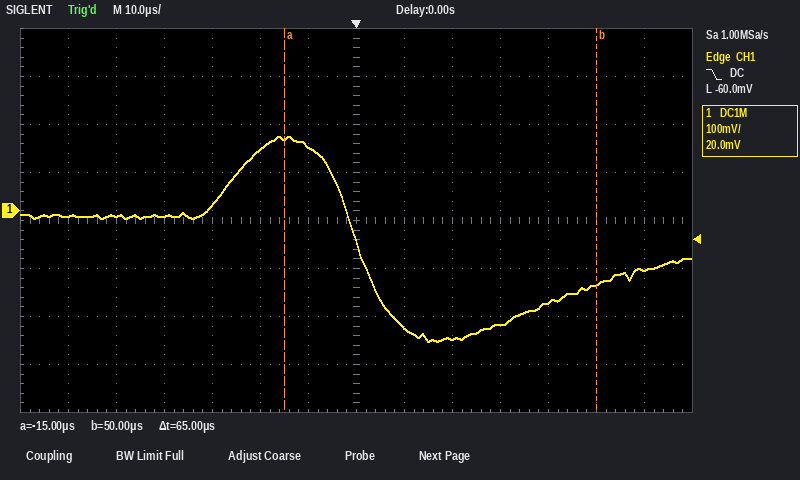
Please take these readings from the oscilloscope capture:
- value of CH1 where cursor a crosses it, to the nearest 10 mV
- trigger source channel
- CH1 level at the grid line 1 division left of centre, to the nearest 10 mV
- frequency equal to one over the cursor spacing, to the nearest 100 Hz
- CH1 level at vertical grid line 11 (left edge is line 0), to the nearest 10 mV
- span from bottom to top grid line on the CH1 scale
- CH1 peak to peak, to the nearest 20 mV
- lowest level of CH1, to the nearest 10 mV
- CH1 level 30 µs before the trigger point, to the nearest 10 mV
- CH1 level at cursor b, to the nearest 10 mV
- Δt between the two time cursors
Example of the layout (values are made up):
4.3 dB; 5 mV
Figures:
150 mV; CH1; 130 mV; 15.4 kHz; -190 mV; 800 mV; 420 mV; -270 mV; 10 mV; -150 mV; 65 µs
